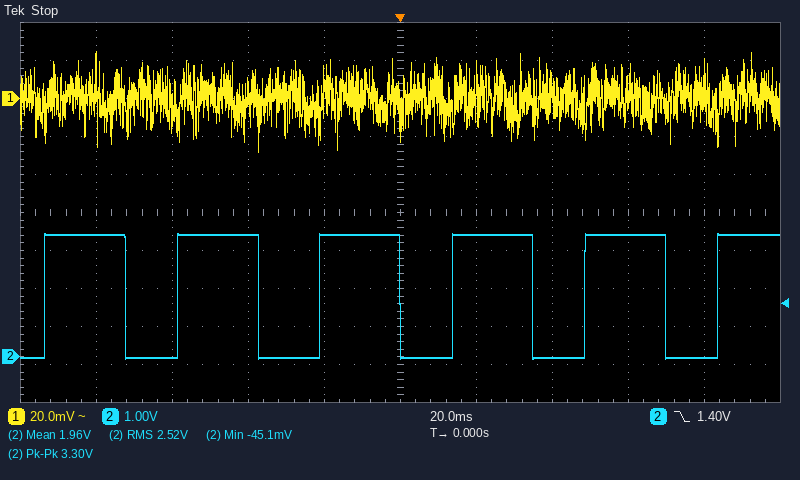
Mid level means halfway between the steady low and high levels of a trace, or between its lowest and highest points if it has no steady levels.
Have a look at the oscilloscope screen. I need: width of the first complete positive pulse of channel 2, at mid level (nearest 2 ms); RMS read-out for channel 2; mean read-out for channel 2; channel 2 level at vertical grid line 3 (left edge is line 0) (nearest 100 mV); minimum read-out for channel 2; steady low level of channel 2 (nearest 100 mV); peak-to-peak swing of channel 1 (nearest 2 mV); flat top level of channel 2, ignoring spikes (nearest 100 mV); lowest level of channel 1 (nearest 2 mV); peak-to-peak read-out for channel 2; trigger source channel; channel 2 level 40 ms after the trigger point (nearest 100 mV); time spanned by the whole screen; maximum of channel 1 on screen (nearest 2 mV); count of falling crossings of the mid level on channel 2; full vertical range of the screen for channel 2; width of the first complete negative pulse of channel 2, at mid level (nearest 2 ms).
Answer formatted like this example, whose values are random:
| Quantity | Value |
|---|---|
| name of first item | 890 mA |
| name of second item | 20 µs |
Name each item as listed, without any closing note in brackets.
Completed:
| Quantity | Value |
|---|---|
| width of the first complete positive pulse of channel 2, at mid level | 22 ms |
| RMS read-out for channel 2 | 2.52 V |
| mean read-out for channel 2 | 1.96 V |
| channel 2 level at vertical grid line 3 (left edge is line 0) | 3.2 V |
| minimum read-out for channel 2 | -45.1 mV |
| steady low level of channel 2 | 0.0 V |
| peak-to-peak swing of channel 1 | 52 mV |
| flat top level of channel 2, ignoring spikes | 3.2 V |
| lowest level of channel 1 | -28 mV |
| peak-to-peak read-out for channel 2 | 3.30 V |
| trigger source channel | channel 2 |
| channel 2 level 40 ms after the trigger point | 0.0 V |
| time spanned by the whole screen | 200 ms |
| maximum of channel 1 on screen | 24 mV |
| count of falling crossings of the mid level on channel 2 | 5 |
| full vertical range of the screen for channel 2 | 10 V |
| width of the first complete negative pulse of channel 2, at mid level | 14 ms |
